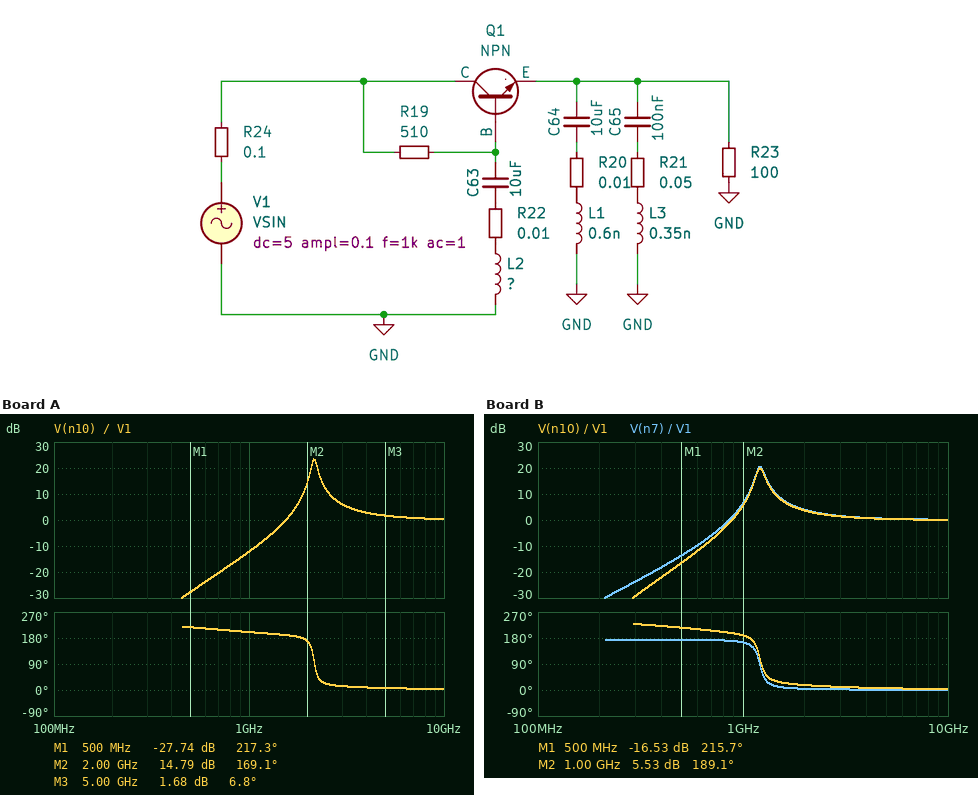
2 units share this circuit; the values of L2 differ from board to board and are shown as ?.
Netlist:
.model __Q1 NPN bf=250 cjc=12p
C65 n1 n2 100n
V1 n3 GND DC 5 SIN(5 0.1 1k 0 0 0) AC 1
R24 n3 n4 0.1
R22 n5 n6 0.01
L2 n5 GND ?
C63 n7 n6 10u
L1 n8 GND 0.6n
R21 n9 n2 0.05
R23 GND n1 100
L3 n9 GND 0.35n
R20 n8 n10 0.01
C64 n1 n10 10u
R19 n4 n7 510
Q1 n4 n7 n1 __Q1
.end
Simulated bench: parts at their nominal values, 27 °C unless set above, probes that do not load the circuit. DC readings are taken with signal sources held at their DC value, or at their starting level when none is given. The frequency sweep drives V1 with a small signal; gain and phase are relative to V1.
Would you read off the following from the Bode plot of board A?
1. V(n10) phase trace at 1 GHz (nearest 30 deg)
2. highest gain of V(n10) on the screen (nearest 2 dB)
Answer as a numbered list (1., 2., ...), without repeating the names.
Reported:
1. 210 deg
2. 24 dB
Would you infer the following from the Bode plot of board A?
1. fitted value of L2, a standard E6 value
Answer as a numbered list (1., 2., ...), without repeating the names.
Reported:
1. 470 pH
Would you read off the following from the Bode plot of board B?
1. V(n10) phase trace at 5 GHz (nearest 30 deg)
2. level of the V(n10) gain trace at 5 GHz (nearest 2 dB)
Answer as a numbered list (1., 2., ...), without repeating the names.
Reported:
1. 0 deg
2. 0 dB
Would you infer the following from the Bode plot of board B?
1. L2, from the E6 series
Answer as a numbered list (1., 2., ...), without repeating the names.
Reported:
1. 1.5 nH
